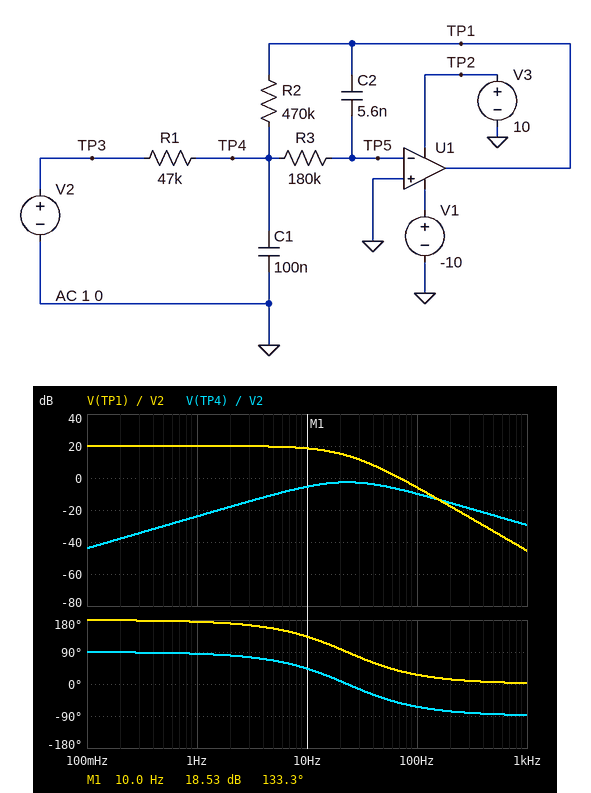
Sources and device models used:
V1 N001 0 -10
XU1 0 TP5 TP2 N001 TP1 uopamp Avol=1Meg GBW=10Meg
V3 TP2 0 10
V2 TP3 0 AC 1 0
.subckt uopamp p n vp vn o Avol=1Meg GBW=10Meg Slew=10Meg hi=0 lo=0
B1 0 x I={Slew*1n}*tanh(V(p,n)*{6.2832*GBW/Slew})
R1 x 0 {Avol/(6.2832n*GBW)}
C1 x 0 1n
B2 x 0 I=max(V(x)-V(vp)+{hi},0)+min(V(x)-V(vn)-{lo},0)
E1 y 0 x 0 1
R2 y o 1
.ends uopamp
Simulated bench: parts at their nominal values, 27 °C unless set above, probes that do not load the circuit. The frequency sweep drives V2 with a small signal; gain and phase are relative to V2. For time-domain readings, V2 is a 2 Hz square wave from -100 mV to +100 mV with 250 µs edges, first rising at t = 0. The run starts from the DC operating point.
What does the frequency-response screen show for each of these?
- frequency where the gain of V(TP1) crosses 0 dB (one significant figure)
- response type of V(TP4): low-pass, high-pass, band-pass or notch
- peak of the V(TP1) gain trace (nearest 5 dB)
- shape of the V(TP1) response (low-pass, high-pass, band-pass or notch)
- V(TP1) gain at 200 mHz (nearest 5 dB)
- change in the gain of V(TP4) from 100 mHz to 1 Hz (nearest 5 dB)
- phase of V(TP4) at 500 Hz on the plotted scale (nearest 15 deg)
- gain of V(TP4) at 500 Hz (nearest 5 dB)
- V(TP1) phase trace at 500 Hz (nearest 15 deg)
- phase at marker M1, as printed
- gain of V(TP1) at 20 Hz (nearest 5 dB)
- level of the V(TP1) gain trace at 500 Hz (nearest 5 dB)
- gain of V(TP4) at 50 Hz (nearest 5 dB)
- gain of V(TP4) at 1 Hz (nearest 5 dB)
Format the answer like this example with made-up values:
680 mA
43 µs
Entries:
70 Hz
band-pass
20 dB
low-pass
20 dB
20 dB
-90 deg
-25 dB
0 deg
133.3 deg
15 dB
-35 dB
-5 dB
-25 dB
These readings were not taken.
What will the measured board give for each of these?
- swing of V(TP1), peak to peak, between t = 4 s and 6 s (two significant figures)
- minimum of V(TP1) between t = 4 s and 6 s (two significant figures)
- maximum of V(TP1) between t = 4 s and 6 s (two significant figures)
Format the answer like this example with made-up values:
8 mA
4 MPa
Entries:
2.0 V
-1.0 V
1.0 V
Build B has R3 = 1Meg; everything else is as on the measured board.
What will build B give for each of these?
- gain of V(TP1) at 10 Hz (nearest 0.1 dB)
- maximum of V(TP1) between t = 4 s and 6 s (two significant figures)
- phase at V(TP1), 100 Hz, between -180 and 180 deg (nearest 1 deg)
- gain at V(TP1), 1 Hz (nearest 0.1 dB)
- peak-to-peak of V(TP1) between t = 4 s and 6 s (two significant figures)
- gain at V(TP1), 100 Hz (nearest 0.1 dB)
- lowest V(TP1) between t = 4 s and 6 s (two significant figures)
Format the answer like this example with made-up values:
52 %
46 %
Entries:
7.9 dB
970 mV
21 deg
19.4 dB
1.9 V
-20.9 dB
-970 mV
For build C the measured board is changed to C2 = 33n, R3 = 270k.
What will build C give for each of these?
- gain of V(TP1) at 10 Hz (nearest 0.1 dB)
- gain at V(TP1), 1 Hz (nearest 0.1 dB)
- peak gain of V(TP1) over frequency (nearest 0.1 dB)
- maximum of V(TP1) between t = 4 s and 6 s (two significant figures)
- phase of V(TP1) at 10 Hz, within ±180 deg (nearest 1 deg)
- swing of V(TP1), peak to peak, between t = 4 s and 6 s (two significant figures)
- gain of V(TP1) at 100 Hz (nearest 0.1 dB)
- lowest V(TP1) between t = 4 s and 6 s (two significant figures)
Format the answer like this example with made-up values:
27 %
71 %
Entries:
2.9 dB
18.3 dB
20.0 dB
810 mV
85 deg
1.6 V
-25.1 dB
-810 mV
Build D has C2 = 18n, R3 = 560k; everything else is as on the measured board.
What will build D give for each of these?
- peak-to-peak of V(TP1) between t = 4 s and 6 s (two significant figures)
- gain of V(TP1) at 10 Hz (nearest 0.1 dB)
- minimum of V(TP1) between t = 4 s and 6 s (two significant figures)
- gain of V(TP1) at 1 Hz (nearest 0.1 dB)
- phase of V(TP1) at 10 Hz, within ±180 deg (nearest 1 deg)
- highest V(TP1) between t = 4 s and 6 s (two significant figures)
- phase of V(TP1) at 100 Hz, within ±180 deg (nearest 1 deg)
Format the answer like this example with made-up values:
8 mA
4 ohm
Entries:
1.6 V
2.4 dB
-790 mV
18.2 dB
83 deg
790 mV
22 deg
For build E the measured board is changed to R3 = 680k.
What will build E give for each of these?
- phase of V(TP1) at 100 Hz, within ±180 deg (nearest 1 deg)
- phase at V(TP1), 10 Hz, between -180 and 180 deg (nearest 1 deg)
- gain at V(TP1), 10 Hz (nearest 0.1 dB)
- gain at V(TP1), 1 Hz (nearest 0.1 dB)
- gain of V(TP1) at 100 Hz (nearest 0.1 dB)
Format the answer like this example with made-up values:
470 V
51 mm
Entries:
22 deg
96 deg
11.0 dB
19.7 dB
-17.5 dB
